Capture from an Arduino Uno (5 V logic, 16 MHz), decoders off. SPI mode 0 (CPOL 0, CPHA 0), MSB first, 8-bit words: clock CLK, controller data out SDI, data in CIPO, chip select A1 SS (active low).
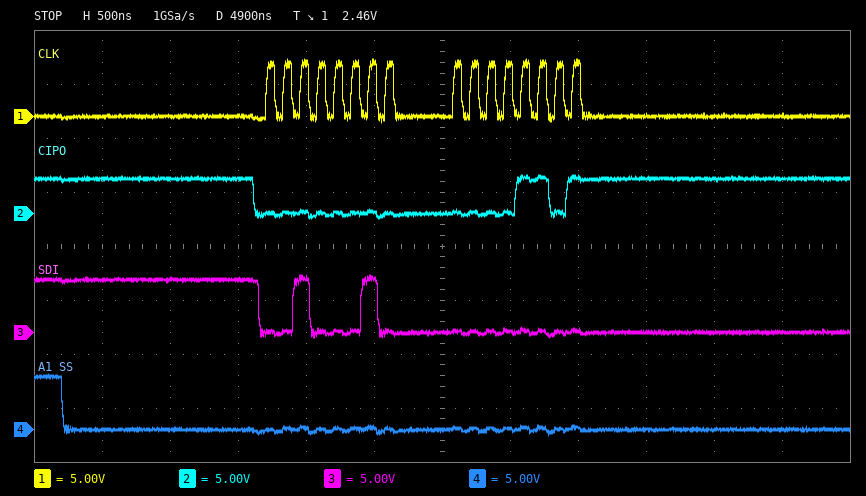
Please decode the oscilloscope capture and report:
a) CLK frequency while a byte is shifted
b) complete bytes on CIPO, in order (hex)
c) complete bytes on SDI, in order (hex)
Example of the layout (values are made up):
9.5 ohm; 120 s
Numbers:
8 MHz; 00 0D; 22 00
